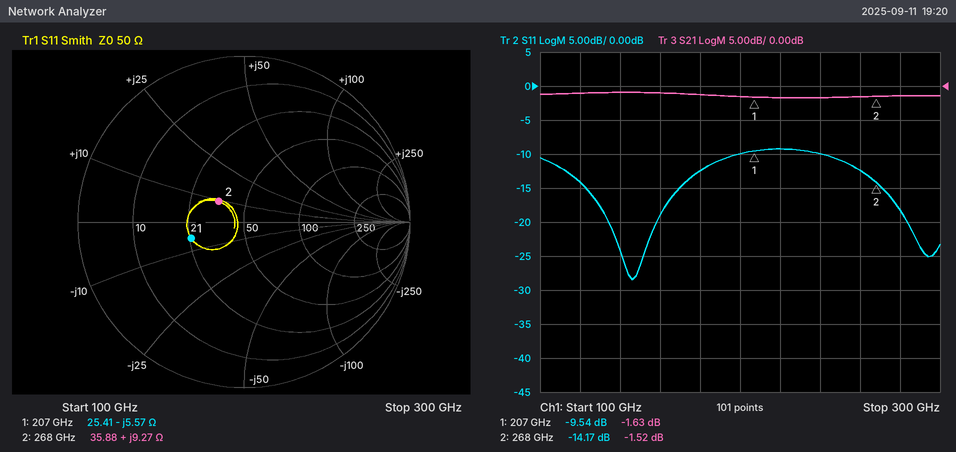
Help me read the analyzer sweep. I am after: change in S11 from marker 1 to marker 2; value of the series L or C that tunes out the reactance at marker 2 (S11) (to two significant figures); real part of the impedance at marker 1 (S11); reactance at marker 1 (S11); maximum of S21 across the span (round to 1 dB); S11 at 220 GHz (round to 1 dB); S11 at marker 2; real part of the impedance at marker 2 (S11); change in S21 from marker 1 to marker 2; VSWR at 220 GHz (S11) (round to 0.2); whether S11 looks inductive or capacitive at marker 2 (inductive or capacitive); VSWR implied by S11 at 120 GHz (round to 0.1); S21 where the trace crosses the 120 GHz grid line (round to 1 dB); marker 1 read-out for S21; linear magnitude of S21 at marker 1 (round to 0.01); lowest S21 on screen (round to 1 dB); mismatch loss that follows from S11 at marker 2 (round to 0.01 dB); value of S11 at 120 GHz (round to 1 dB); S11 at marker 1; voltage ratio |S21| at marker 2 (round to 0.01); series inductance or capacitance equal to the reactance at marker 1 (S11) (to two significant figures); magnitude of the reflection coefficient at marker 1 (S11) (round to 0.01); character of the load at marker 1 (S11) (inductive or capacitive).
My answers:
-4.63 dB
64 fF
25.41 Ω
-5.57 Ω
-1 dB
-9 dB
-14.17 dB
35.88 Ω
0.11 dB
2.0
inductive
1.5
-1 dB
-1.63 dB
0.83
-2 dB
0.17 dB
-14 dB
-9.54 dB
0.84
140 fF
0.33
capacitive
